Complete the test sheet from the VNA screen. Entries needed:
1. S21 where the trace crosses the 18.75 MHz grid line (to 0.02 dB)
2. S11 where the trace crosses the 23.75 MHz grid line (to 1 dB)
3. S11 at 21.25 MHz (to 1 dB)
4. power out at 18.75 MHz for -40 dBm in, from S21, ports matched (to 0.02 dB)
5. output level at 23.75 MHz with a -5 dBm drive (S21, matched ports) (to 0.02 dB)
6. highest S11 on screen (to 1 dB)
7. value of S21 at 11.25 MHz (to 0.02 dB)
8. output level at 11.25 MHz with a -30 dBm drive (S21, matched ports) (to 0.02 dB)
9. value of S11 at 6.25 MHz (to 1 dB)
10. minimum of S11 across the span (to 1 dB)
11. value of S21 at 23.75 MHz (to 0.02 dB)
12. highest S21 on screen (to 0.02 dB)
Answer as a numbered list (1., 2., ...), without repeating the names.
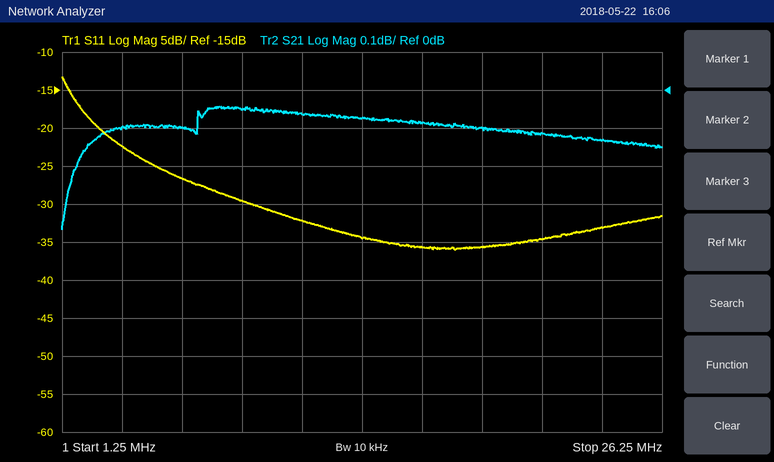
1. -0.10 dB
2. -33 dB
3. -35 dB
4. -40.10 dBm
5. -5.14 dBm
6. -13 dB
7. -0.06 dB
8. -30.06 dBm
9. -27 dB
10. -36 dB
11. -0.14 dB
12. -0.04 dB
